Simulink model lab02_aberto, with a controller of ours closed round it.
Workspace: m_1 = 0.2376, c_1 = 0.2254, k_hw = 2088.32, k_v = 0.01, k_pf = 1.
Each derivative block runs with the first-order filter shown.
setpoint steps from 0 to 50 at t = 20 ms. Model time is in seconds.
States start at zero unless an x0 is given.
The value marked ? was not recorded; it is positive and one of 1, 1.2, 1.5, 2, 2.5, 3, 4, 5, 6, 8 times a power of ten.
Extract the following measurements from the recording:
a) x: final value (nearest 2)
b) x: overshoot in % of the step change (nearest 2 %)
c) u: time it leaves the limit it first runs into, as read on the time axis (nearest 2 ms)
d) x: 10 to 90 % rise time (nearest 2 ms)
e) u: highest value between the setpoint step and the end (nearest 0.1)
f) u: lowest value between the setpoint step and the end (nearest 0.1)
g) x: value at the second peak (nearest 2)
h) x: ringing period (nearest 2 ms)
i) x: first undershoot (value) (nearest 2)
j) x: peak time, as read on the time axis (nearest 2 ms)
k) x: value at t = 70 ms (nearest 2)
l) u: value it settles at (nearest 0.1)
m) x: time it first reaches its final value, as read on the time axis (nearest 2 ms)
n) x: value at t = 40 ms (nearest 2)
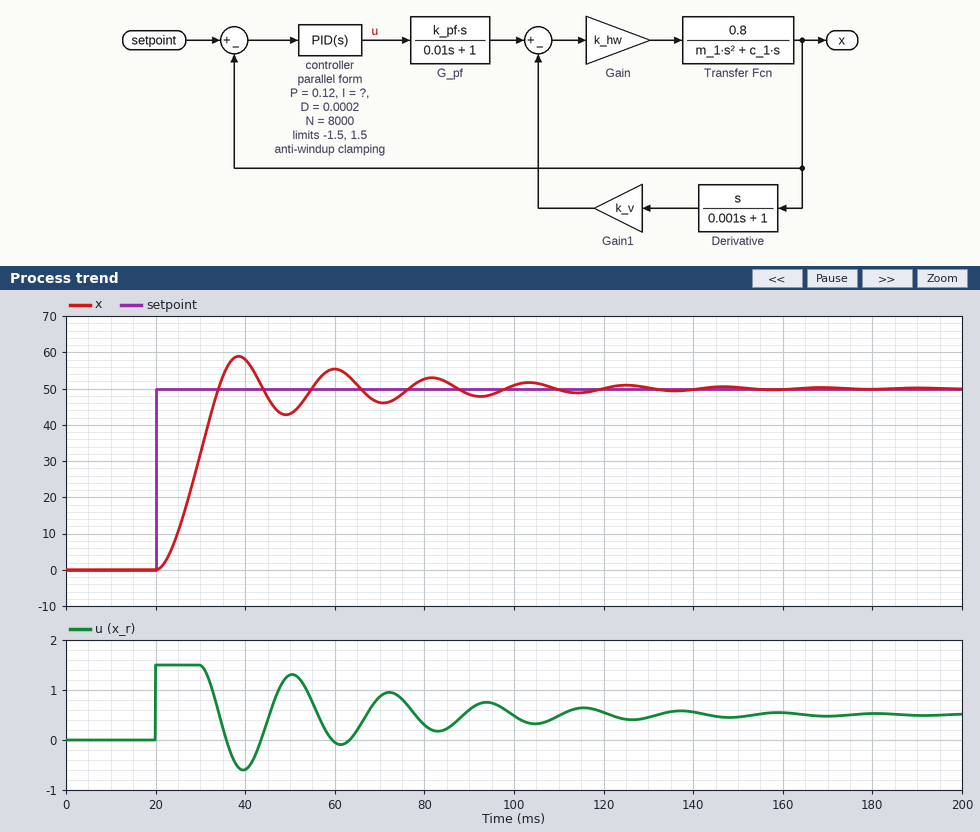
50
18 %
30 ms
10 ms
1.5
-0.6
56
22 ms
42
38 ms
46
0.5
34 ms
58
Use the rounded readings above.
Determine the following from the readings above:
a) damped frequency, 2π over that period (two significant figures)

0.29 rad/ms
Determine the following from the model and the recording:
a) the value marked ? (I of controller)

30
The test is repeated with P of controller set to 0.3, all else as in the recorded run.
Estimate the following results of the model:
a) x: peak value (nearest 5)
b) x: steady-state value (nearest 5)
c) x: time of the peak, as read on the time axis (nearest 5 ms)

55
50
35 ms
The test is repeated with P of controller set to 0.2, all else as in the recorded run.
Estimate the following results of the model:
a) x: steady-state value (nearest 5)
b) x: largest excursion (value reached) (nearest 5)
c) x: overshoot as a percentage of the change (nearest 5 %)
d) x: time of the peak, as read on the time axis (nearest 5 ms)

50
55
10 %
35 ms
